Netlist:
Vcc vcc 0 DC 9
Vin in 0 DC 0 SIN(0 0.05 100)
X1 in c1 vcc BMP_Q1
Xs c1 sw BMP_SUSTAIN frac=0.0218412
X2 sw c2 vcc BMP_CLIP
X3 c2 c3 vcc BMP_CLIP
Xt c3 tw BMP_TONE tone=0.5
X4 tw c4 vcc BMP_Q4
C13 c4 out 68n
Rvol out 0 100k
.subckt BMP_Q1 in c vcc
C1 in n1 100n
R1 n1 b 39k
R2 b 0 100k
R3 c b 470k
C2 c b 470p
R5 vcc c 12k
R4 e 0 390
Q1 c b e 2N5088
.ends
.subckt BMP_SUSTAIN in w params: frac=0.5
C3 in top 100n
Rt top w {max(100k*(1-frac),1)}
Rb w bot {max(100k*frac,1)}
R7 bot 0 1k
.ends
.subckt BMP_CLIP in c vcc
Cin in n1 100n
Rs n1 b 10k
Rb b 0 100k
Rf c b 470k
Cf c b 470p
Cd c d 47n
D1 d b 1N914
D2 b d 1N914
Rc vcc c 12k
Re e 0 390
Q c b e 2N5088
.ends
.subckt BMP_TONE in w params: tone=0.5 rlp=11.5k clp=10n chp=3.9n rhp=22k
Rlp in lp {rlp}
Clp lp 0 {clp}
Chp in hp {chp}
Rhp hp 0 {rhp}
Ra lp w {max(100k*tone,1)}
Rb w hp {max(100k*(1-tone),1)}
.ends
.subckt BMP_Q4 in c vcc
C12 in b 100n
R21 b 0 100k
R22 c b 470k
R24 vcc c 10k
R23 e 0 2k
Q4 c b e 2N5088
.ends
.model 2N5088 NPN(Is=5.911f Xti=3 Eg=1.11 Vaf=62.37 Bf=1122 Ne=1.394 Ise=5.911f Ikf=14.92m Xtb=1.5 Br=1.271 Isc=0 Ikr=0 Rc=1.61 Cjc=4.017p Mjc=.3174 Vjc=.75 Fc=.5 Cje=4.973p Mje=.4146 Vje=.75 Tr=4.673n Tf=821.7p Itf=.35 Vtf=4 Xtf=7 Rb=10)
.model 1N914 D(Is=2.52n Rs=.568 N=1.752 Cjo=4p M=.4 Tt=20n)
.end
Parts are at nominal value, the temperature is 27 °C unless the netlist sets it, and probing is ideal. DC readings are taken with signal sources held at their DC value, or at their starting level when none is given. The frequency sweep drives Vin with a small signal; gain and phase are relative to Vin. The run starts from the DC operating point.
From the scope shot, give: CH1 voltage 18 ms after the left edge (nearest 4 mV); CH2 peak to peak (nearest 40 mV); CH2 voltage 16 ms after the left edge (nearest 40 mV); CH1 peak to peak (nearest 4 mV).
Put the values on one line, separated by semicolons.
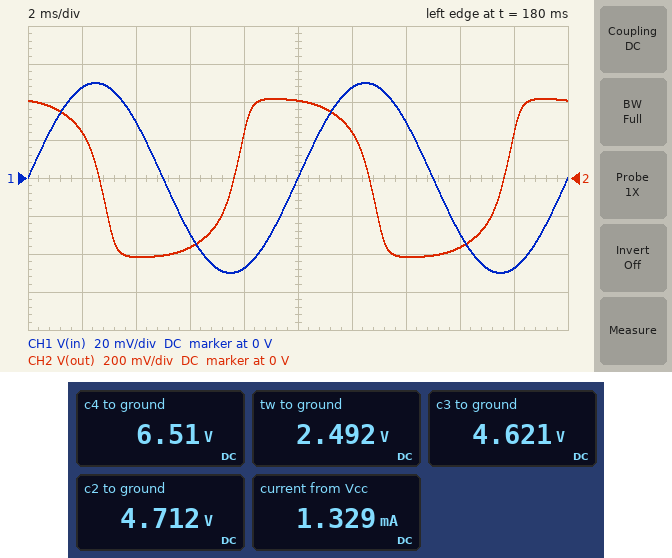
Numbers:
-48 mV; 840 mV; -360 mV; 100 mV
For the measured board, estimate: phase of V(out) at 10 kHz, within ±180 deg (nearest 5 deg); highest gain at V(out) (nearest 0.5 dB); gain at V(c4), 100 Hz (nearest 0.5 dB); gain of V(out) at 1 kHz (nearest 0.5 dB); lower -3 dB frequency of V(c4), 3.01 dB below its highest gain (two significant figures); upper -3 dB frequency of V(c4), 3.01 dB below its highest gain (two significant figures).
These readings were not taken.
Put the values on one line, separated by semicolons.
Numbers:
135 deg; 29.5 dB; 28.0 dB; 23.0 dB; 74 Hz; 650 Hz
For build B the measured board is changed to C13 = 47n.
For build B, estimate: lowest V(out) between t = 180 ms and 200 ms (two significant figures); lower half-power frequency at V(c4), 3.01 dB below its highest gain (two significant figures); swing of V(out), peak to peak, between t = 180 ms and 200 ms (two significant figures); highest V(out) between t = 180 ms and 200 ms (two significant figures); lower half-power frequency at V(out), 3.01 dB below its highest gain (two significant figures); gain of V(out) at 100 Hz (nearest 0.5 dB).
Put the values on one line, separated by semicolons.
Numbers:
-430 mV; 73 Hz; 860 mV; 430 mV; 80 Hz; 27.5 dB
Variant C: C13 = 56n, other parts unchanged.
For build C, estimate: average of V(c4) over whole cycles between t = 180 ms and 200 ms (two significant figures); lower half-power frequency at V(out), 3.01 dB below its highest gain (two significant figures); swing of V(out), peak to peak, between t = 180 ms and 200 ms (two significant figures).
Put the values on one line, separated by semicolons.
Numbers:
6.5 V; 79 Hz; 850 mV
